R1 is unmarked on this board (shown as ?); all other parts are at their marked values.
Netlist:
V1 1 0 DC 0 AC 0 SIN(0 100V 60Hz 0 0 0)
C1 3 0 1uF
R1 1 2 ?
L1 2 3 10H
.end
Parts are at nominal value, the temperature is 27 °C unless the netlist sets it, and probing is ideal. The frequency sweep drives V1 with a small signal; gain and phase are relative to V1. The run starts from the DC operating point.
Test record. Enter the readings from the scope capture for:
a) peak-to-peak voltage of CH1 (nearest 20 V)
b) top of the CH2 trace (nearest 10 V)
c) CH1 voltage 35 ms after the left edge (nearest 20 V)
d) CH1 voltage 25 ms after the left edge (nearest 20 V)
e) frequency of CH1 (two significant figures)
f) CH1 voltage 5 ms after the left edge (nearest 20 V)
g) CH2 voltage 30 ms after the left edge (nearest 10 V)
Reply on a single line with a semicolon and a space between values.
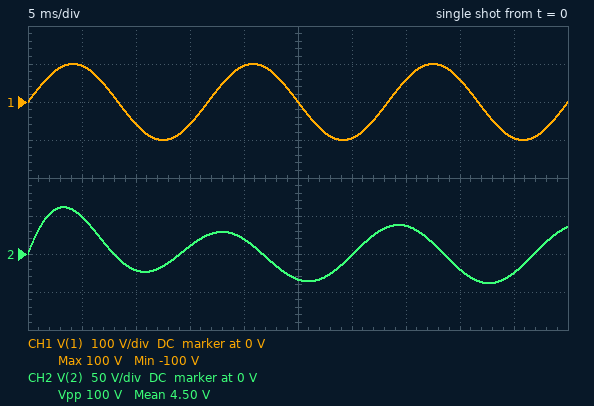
200 V; 60 V; 60 V; 0 V; 60 Hz; 100 V; 0 V
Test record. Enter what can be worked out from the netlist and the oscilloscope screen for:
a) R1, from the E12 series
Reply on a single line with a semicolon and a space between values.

2.7 kΩ
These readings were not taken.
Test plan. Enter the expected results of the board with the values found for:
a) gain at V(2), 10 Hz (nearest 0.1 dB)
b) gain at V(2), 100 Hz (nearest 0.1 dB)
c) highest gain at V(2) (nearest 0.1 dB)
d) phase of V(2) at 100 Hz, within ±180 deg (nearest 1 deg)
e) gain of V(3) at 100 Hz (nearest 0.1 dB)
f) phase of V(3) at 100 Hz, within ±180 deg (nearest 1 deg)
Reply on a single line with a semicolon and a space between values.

-0.1 dB; -1.2 dB; 0 dB; 30 deg; -10.6 dB; -150 deg
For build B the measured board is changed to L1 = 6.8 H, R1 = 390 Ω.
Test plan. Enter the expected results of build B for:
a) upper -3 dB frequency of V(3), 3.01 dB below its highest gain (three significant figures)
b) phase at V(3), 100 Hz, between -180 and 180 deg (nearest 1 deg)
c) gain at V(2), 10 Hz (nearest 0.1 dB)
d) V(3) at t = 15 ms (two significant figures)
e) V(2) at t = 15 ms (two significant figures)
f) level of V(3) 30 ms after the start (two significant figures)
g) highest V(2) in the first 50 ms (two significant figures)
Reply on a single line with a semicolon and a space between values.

65.1 Hz; -172 deg; 0 dB; -220 V; -41 V; -180 V; 89 V
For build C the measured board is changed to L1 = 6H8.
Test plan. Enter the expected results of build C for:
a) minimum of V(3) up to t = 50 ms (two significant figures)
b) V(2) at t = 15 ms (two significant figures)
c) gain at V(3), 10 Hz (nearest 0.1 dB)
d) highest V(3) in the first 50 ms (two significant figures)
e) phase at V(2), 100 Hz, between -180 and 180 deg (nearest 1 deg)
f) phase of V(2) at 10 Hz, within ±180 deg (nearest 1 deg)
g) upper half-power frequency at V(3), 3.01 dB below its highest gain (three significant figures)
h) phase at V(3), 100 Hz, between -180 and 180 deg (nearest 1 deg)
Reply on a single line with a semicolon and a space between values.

-98 V; -8.5 V; 0.1 dB; 98 V; 45 deg; -10 deg; 70.9 Hz; -135 deg
